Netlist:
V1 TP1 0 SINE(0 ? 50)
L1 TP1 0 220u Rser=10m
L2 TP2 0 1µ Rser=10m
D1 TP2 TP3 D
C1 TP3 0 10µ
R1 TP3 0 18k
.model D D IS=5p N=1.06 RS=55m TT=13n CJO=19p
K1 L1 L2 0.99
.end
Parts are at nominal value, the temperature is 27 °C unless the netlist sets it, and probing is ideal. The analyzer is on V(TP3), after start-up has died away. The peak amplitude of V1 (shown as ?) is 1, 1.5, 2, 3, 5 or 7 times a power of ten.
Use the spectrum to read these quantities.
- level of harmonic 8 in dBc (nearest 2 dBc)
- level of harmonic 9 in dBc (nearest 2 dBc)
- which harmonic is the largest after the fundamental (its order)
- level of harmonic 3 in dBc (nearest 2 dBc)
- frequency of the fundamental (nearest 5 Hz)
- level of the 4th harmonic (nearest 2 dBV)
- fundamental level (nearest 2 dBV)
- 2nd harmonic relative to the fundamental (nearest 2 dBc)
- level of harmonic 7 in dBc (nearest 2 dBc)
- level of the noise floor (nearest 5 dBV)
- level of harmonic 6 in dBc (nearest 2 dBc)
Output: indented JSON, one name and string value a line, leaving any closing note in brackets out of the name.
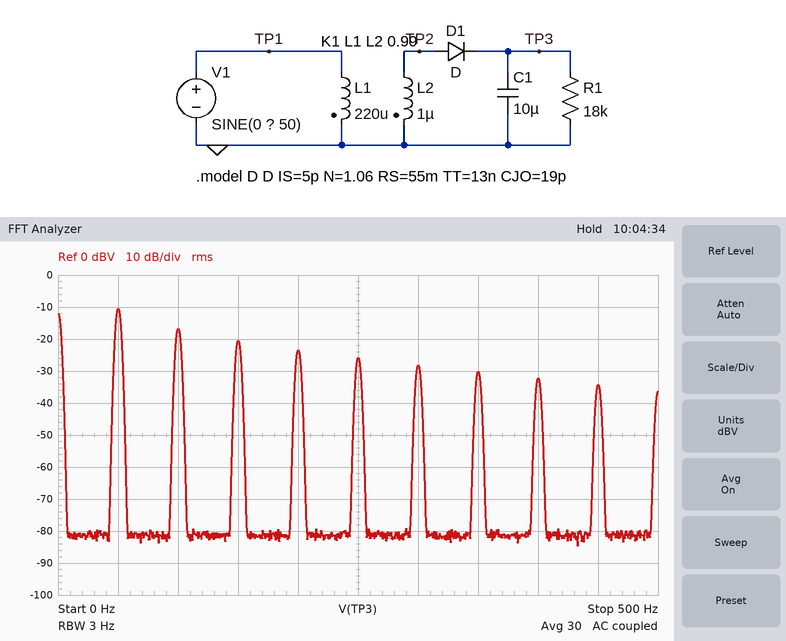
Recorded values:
{
  "level of harmonic 8 in dBc": "-22 dBc",
  "level of harmonic 9 in dBc": "-24 dBc",
  "which harmonic is the largest after the fundamental": "2",
  "level of harmonic 3 in dBc": "-10 dBc",
  "frequency of the fundamental": "50 Hz",
  "level of the 4th harmonic": "-24 dBV",
  "fundamental level": "-10 dBV",
  "2nd harmonic relative to the fundamental": "-6 dBc",
  "level of harmonic 7 in dBc": "-20 dBc",
  "level of the noise floor": "-80 dBV",
  "level of harmonic 6 in dBc": "-18 dBc"
}
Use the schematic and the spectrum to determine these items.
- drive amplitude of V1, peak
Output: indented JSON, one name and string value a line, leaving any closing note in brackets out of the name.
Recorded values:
{
  "drive amplitude of V1, peak": "200 V"
}
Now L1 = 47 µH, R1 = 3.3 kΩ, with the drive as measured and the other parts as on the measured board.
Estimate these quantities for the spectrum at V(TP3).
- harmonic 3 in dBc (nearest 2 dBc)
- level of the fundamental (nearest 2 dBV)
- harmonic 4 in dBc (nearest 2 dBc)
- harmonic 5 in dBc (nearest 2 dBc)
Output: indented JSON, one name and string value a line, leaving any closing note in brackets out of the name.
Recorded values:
{
  "harmonic 3 in dBc": "-12 dBc",
  "level of the fundamental": "8 dBV",
  "harmonic 4 in dBc": "-16 dBc",
  "harmonic 5 in dBc": "-20 dBc"
}
